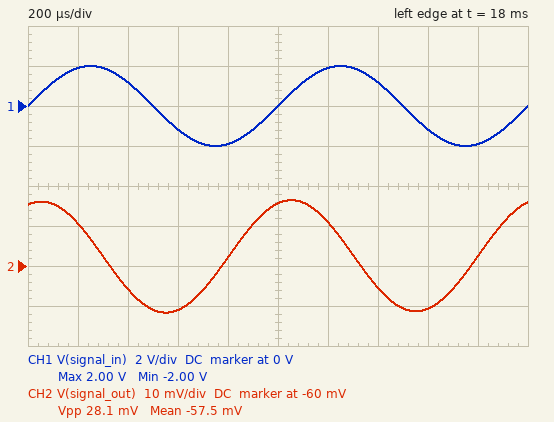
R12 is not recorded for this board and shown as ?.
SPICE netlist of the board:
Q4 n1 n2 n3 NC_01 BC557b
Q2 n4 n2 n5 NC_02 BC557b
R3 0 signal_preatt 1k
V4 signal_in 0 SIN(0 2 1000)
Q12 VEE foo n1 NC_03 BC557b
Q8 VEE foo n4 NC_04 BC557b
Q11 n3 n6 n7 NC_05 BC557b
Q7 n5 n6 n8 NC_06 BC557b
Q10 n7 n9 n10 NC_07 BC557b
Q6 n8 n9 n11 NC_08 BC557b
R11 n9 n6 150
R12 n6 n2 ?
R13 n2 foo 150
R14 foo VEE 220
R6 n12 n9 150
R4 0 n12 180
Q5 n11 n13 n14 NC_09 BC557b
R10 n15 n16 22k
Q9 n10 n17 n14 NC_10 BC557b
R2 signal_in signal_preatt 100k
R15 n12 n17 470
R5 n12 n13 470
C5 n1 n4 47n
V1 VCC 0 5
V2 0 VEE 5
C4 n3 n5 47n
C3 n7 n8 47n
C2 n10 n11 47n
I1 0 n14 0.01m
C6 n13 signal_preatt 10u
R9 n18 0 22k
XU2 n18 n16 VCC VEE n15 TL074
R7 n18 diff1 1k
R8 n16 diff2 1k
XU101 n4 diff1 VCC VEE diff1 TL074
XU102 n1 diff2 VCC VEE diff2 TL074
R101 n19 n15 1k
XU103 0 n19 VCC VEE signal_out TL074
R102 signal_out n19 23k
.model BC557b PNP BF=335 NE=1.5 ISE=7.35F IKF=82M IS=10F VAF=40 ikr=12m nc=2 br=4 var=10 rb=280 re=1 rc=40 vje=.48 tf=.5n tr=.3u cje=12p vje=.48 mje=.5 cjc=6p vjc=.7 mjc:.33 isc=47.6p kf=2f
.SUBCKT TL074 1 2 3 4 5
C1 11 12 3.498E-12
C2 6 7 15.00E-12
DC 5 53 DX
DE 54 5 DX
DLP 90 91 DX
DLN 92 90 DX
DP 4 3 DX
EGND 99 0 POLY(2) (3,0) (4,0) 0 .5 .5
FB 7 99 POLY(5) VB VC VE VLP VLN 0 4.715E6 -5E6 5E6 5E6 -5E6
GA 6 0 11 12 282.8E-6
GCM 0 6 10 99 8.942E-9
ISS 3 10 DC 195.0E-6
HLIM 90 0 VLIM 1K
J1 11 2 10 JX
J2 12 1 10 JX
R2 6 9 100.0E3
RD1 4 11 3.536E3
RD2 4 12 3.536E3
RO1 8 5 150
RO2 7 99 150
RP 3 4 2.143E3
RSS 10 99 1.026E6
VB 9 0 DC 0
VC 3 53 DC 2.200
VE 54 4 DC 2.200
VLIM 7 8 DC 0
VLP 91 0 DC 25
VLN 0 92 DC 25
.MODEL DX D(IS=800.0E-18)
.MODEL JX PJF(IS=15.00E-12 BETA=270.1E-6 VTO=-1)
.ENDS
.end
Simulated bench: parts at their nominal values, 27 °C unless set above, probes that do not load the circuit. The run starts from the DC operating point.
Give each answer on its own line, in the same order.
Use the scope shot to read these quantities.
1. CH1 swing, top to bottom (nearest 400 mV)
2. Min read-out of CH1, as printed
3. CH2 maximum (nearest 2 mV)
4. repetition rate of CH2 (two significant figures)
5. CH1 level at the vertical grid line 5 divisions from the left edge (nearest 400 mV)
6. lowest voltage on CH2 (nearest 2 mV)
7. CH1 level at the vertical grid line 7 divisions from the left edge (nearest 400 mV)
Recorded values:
4.0 V
-2.00 V
-44 mV
1.0 kHz
0 V
-72 mV
1.2 V
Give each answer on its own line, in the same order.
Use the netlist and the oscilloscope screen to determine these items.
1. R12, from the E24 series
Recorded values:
180 Ω
